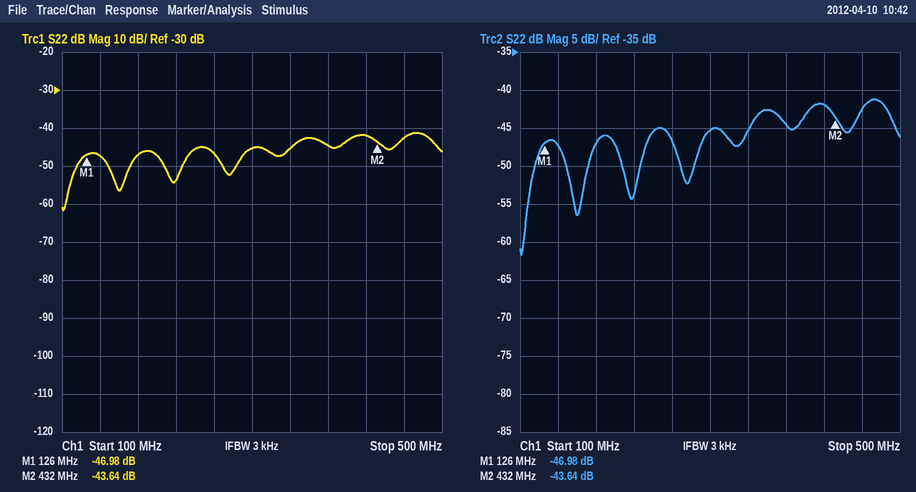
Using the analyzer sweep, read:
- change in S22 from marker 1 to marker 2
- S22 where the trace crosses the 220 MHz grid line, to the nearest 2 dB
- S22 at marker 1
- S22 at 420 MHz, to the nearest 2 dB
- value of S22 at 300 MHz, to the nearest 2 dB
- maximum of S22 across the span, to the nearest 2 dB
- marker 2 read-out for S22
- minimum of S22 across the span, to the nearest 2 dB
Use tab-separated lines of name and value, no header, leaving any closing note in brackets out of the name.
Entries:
change in S22 from marker 1 to marker 2	3.34 dB
S22 where the trace crosses the 220 MHz grid line, to the nearest 2 dB	-54 dB
S22 at marker 1	-46.98 dB
S22 at 420 MHz, to the nearest 2 dB	-42 dB
value of S22 at 300 MHz, to the nearest 2 dB	-46 dB
maximum of S22 across the span, to the nearest 2 dB	-42 dB
marker 2 read-out for S22	-43.64 dB
minimum of S22 across the span, to the nearest 2 dB	-62 dB
